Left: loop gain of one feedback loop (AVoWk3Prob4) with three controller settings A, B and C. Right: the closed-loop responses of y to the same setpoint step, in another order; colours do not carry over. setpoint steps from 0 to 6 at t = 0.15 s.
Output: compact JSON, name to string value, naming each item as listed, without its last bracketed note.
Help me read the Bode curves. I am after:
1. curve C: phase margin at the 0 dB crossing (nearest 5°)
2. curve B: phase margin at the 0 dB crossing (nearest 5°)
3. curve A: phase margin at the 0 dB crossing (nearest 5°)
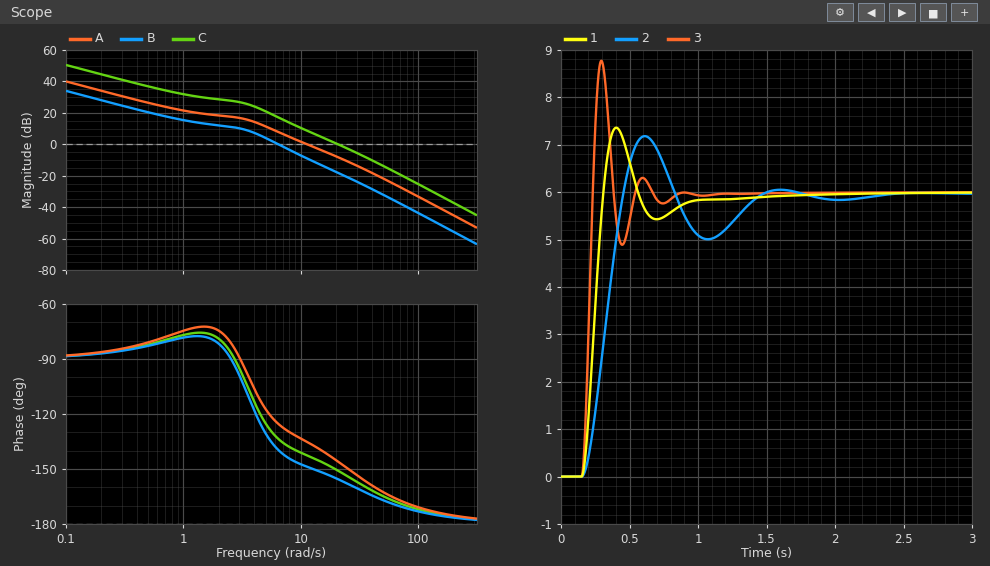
{"curve C: phase margin at the 0 dB crossing": "30°", "curve B: phase margin at the 0 dB crossing": "40°", "curve A: phase margin at the 0 dB crossing": "45°"}
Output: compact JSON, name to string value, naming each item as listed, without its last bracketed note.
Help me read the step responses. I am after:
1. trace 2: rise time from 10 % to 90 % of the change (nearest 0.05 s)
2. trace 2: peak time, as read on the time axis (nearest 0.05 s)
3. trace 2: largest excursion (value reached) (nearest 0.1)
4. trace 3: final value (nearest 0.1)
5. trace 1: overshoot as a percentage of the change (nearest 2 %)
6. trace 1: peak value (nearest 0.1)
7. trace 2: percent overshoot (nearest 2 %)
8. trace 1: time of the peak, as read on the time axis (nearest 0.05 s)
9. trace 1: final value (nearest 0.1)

{"trace 2: rise time from 10 % to 90 % of the change": "0.20 s", "trace 2: peak time, as read on the time axis": "0.60 s", "trace 2: largest excursion (value reached)": "7.2", "trace 3: final value": "6.0", "trace 1: overshoot as a percentage of the change": "22 %", "trace 1: peak value": "7.4", "trace 2: percent overshoot": "20 %", "trace 1: time of the peak, as read on the time axis": "0.40 s", "trace 1: final value": "6.0"}
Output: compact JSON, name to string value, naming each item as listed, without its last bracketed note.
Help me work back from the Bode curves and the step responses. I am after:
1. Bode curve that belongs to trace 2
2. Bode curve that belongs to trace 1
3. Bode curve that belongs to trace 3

{"Bode curve that belongs to trace 2": "B", "Bode curve that belongs to trace 1": "A", "Bode curve that belongs to trace 3": "C"}
